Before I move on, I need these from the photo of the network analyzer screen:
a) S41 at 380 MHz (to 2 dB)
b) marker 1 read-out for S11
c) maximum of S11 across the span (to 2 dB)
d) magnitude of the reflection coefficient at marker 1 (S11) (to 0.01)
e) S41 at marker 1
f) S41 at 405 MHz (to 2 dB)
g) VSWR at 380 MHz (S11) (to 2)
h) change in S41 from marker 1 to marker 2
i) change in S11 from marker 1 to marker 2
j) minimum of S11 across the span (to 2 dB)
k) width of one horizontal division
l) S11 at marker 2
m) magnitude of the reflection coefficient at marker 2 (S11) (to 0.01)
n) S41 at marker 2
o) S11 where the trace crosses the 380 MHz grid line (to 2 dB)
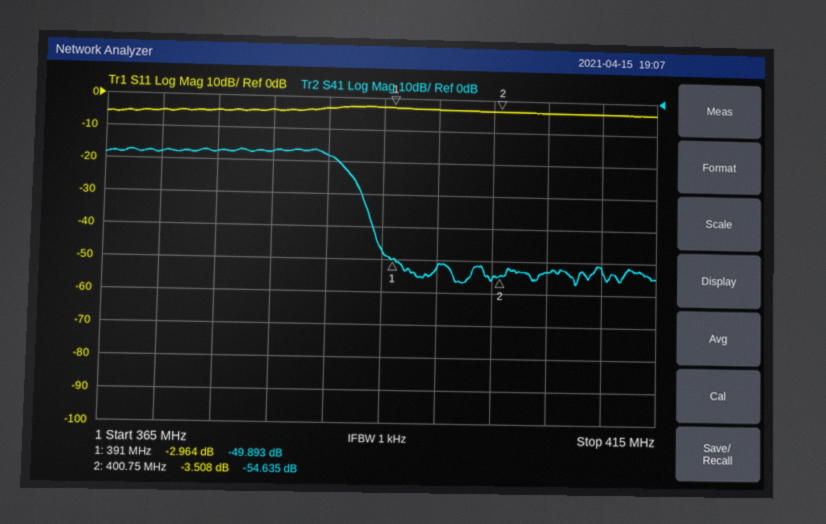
-18 dB
-2.964 dB
-2 dB
0.71
-49.893 dB
-54 dB
4
-4.742 dB
-0.544 dB
-6 dB
5 MHz
-3.508 dB
0.67
-54.635 dB
-4 dB
